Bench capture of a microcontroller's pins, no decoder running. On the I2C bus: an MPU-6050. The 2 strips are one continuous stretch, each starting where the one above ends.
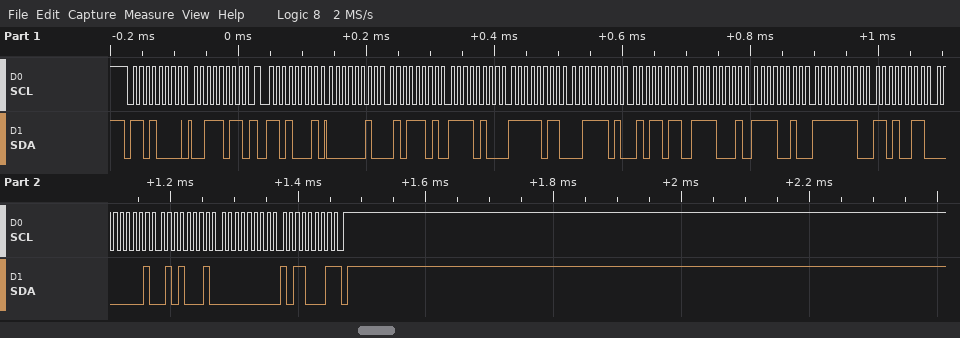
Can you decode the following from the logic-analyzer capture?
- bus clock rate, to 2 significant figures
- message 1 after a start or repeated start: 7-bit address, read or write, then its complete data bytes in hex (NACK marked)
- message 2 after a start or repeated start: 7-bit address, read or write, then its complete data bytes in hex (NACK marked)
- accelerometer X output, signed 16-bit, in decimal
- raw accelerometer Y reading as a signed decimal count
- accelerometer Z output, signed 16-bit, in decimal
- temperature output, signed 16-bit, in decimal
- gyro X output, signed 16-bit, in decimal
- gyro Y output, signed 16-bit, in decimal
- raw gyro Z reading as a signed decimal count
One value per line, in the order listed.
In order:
100 kHz
0x68 write: 3B
0x68 read: 02 5D F4 FB 3D 5B F1 F2 FE D3 01 51 00 B1 NACK
605
-2821
15707
-3598
-301
337
177
